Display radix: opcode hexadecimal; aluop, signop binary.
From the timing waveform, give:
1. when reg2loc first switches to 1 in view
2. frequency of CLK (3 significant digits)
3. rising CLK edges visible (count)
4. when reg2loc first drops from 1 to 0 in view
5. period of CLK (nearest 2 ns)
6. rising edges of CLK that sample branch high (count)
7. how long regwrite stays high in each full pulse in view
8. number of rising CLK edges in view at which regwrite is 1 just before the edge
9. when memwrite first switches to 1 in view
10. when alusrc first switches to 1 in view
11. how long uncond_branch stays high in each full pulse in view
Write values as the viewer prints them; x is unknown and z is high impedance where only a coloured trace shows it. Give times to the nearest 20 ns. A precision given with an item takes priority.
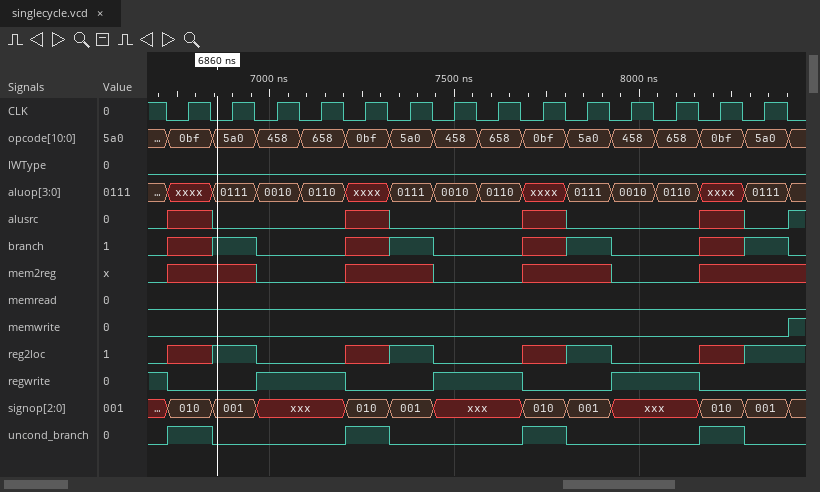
6840 ns
8.33 MHz
14
6960 ns
120 ns
4
240 ns, 240 ns, 240 ns
6
8400 ns
8400 ns
120 ns, 120 ns, 120 ns, 120 ns
